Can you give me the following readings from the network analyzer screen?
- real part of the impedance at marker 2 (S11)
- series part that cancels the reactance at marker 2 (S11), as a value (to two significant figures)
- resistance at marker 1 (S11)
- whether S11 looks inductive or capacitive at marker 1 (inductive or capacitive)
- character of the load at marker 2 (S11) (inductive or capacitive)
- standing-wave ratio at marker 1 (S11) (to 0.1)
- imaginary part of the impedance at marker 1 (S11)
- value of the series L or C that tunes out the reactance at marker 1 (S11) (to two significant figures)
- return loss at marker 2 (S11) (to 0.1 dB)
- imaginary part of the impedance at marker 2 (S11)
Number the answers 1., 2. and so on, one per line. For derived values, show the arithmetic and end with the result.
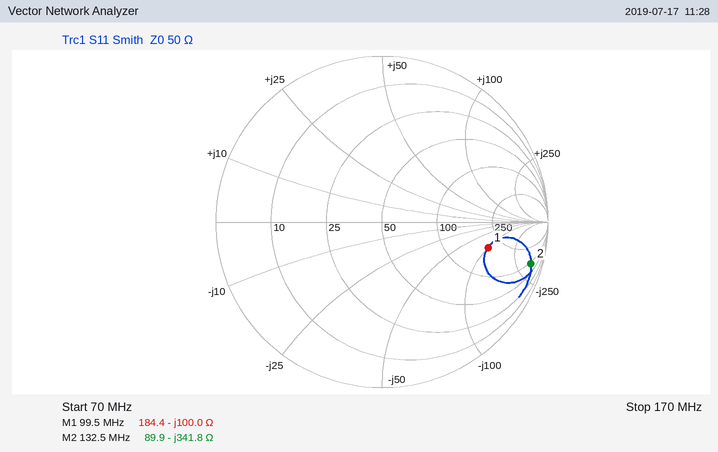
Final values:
1. 89.9 Ω
2. L = 341.8 Ω/(2π × 132.5 MHz) ≈ 411 nH, so 410 nH to two significant figures
3. 184.4 Ω
4. capacitive
5. capacitive
6. 4.8
7. -100.0 Ω
8. L = 100 Ω/(2π × 99.5 MHz) ≈ 160 nH
9. 0.6 dB
10. -341.8 Ω
